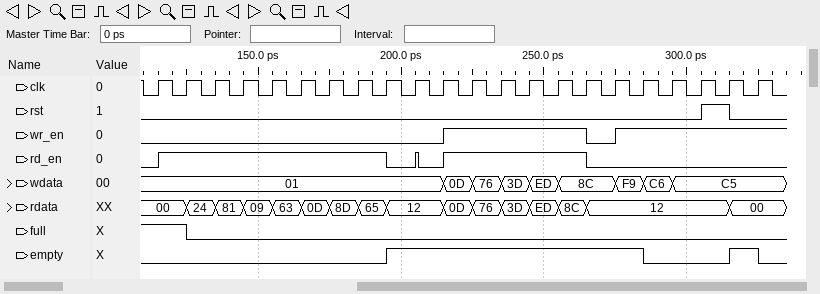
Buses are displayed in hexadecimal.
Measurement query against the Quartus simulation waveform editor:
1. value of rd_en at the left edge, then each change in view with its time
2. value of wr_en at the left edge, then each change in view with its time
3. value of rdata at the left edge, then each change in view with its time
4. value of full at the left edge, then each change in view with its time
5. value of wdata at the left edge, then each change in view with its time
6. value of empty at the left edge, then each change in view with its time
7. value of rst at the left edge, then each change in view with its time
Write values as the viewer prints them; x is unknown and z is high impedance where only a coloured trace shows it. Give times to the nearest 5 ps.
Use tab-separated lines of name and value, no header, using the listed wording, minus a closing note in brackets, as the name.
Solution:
value of rd_en at the left edge, then each change in view with its time	0, 1 at 115 ps, 0 at 195 ps, 1 at 205 ps, 0 at 205 ps, 1 at 215 ps, 0 at 265 ps
value of wr_en at the left edge, then each change in view with its time	0, 1 at 215 ps, 0 at 265 ps, 1 at 275 ps
value of rdata at the left edge, then each change in view with its time	00, 24 at 125 ps, 81 at 135 ps, 09 at 145 ps, 63 at 155 ps, 0D at 165 ps, 8D at 175 ps, 65 at 185 ps, 12 at 195 ps, 0D at 215 ps, 76 at 225 ps, 3D at 235 ps, ED at 245 ps, 8C at 255 ps, 12 at 265 ps, 00 at 315 ps
value of full at the left edge, then each change in view with its time	1, 0 at 125 ps
value of wdata at the left edge, then each change in view with its time	01, 0D at 215 ps, 76 at 225 ps, 3D at 235 ps, ED at 245 ps, 8C at 255 ps, F9 at 275 ps, C6 at 285 ps, C5 at 295 ps
value of empty at the left edge, then each change in view with its time	0, 1 at 195 ps, 0 at 285 ps, 1 at 315 ps, 0 at 325 ps
value of rst at the left edge, then each change in view with its time	0, 1 at 305 ps, 0 at 315 ps
